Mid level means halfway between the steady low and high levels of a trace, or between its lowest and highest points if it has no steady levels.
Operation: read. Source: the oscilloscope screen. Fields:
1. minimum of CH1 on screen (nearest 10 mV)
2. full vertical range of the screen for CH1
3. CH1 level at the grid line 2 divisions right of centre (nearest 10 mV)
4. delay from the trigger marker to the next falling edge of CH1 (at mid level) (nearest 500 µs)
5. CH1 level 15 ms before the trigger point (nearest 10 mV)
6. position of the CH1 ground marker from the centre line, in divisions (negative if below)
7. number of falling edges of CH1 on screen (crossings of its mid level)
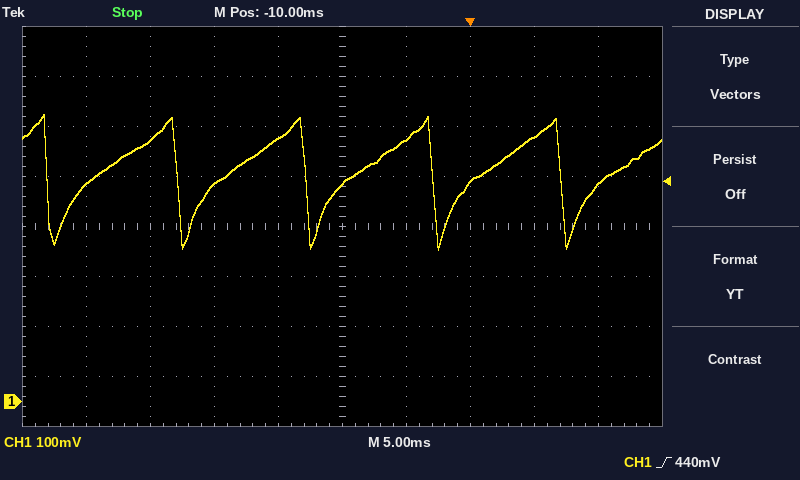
300 mV
800 mV
440 mV
7.0 ms
530 mV
-3.5 div
5
